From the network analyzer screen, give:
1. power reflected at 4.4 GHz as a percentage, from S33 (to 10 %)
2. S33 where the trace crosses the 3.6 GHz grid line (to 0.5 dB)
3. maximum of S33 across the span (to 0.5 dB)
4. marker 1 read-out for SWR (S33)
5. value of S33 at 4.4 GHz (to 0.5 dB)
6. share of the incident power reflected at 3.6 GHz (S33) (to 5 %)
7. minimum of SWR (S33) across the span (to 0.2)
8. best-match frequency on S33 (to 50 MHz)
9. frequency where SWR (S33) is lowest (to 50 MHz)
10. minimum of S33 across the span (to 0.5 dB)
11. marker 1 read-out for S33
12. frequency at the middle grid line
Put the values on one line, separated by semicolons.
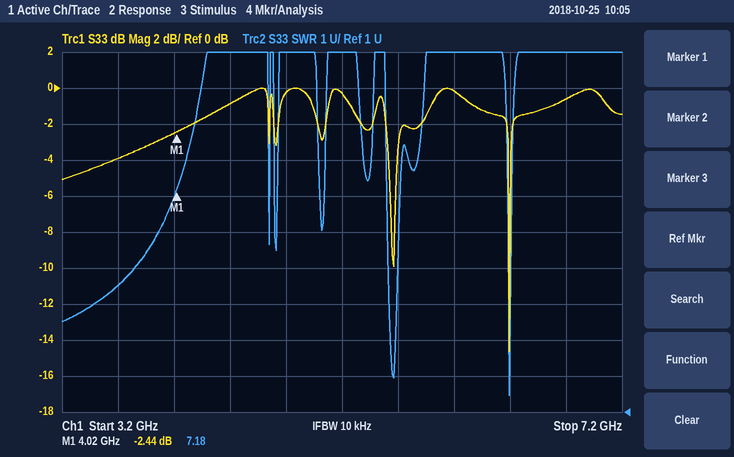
80 %; -4.0 dB; 0.0 dB; 7.18; -1.0 dB; 40 %; 1.4; 6.40 GHz; 6.40 GHz; -14.5 dB; -2.44 dB; 5.2 GHz
